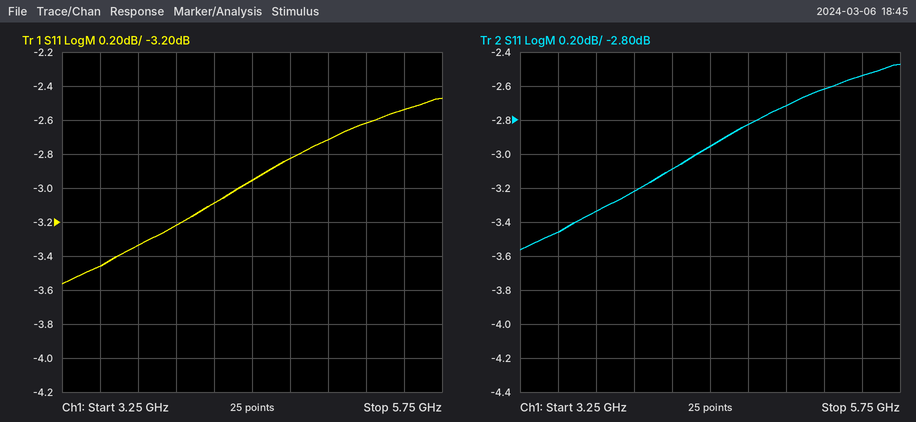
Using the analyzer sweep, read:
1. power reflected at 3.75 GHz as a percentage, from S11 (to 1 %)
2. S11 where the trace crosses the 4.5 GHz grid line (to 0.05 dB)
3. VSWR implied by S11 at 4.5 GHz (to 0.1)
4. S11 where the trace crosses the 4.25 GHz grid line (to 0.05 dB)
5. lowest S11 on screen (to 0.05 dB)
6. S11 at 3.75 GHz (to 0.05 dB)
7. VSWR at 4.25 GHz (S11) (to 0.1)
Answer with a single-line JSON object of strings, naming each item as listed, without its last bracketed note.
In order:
{"power reflected at 3.75 GHz as a percentage, from S11": "46 %", "S11 where the trace crosses the 4.5 GHz grid line": "-2.95 dB", "VSWR implied by S11 at 4.5 GHz": "5.9", "S11 where the trace crosses the 4.25 GHz grid line": "-3.10 dB", "lowest S11 on screen": "-3.55 dB", "S11 at 3.75 GHz": "-3.35 dB", "VSWR at 4.25 GHz (S11)": "5.7"}
